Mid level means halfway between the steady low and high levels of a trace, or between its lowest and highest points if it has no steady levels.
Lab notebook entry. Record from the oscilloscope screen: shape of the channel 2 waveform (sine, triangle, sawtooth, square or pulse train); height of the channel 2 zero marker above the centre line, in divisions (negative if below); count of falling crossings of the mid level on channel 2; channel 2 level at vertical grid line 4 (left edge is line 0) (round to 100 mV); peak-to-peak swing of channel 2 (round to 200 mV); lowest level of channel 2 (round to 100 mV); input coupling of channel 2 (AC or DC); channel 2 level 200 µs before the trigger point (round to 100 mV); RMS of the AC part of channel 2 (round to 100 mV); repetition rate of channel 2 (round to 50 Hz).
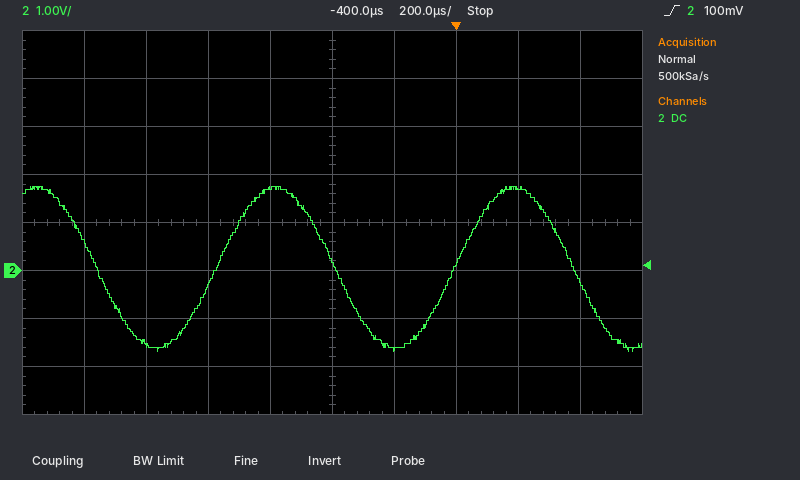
sine
-1.0 div
3
1.7 V
3.4 V
-1.7 V
DC
-1.6 V
1.2 V
1.30 kHz
